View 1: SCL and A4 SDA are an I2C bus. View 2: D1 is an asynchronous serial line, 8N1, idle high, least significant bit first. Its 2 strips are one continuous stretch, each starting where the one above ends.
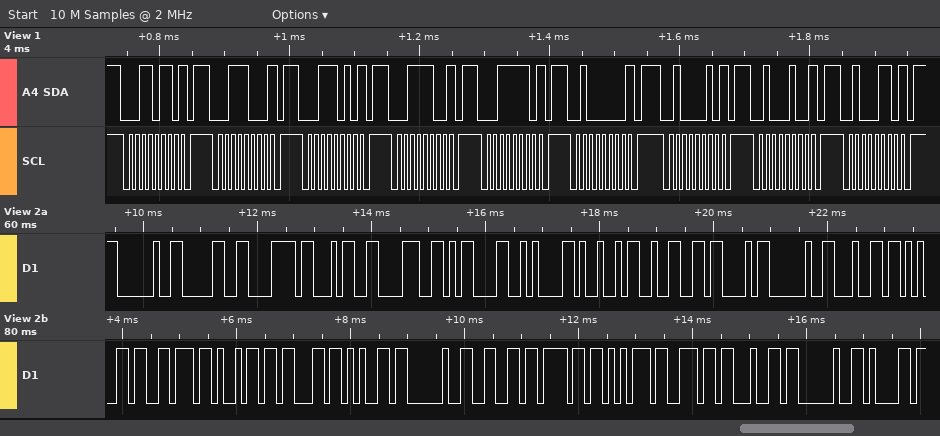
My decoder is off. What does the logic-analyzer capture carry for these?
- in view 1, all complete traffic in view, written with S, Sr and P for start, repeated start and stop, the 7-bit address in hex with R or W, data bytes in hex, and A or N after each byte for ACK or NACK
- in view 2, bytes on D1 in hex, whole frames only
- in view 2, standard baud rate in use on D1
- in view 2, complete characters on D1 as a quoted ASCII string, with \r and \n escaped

S 1BW N P S 1CW N P S 1DW N P S 1EW N P S 1FW N P S 20W N P S 21W N P S 22W N P S 23W N P
20 30 78 34 38 0D 0A 49 32 43 20 64 65 76 69 63 65 20 66 6F 75 6E 64 20 61
9600 baud
" 0x48\r\nI2C device found a"
